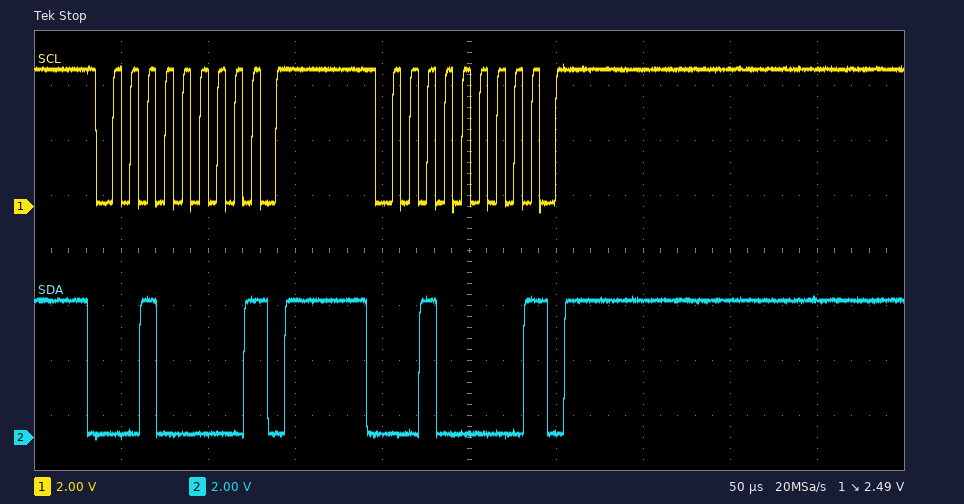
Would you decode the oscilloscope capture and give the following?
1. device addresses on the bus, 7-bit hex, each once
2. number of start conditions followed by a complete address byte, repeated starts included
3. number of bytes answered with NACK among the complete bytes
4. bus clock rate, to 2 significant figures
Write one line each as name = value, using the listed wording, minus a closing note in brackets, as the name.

device addresses on the bus, 7-bit hex, each once = 0x10
number of start conditions followed by a complete address byte, repeated starts included = 2
number of bytes answered with NACK among the complete bytes = 2
bus clock rate, to 2 significant figures = 100 kHz
